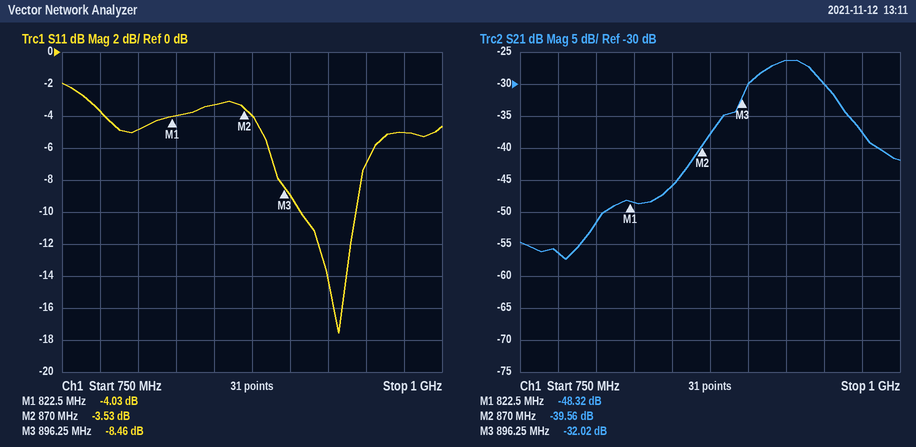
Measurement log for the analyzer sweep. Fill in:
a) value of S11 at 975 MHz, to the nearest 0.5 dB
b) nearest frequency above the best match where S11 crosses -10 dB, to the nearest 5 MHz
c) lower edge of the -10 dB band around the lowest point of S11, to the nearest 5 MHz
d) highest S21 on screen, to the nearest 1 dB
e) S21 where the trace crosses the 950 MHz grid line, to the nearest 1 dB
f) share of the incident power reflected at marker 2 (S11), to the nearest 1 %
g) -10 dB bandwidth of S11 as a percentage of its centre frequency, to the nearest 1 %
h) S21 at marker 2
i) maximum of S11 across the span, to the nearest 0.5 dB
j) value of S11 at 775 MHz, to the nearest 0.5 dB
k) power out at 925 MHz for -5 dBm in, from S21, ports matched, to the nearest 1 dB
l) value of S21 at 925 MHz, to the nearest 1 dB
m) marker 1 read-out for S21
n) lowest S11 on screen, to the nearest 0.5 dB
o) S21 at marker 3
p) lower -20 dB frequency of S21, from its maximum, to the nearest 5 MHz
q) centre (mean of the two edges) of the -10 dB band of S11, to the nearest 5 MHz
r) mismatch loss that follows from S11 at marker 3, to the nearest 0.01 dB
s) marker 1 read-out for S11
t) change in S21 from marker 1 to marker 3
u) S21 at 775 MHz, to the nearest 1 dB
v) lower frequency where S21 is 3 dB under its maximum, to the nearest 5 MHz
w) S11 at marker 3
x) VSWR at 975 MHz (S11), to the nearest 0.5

-5.0 dB
945 MHz
905 MHz
-26 dB
-30 dB
44 %
4 %
-39.56 dB
-2.0 dB
-3.5 dB
-31 dBm
-26 dB
-48.32 dB
-17.5 dB
-32.02 dB
850 MHz
925 MHz
0.67 dB
-4.03 dB
16.30 dB
-56 dB
905 MHz
-8.46 dB
3.5
